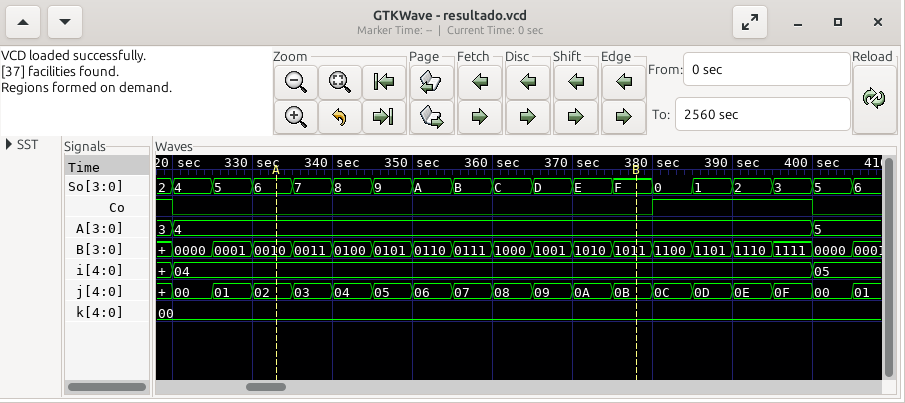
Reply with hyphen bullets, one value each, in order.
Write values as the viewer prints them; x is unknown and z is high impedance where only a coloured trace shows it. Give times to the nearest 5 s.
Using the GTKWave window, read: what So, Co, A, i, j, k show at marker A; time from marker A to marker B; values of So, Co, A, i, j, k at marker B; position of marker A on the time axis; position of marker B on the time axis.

- So=6, Co=0, A=4, i=04, j=02, k=00
- 45 s
- So=F, Co=0, A=4, i=04, j=0B, k=00
- 335 s
- 380 s
